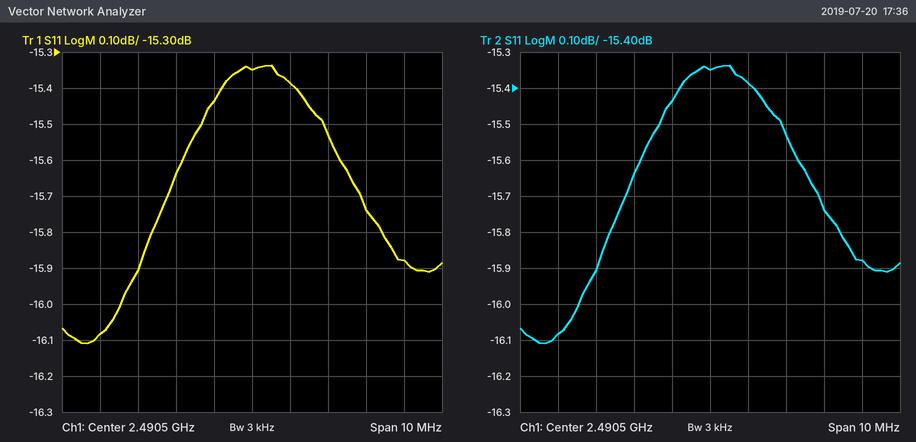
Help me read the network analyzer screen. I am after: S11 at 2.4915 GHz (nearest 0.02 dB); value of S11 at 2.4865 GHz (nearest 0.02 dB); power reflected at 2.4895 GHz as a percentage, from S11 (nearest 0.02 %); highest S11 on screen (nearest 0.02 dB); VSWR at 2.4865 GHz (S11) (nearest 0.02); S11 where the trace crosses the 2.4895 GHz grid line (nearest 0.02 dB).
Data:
-15.38 dB
-16.08 dB
2.86 %
-15.34 dB
1.38
-15.44 dB
